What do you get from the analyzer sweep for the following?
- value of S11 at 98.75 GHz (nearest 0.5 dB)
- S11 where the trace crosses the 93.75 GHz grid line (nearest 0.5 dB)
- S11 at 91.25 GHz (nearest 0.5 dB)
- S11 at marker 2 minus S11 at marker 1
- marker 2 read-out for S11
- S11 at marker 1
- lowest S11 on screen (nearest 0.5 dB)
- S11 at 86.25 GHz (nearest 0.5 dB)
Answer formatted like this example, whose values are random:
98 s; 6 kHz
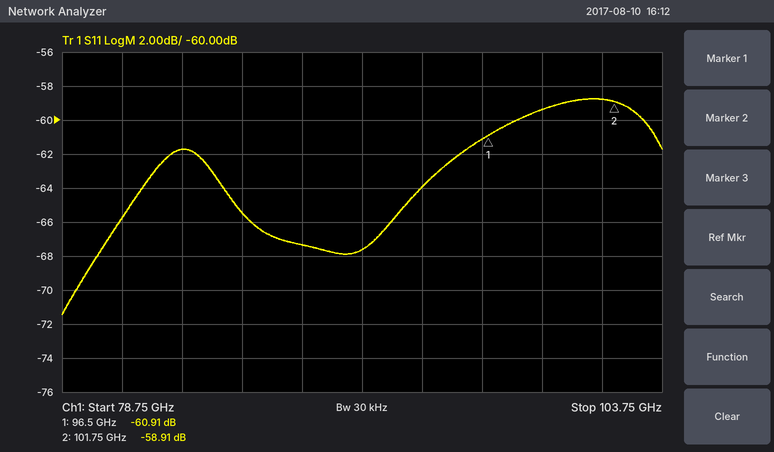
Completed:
-59.5 dB; -64.0 dB; -67.5 dB; 2.00 dB; -58.91 dB; -60.91 dB; -71.5 dB; -65.5 dB
